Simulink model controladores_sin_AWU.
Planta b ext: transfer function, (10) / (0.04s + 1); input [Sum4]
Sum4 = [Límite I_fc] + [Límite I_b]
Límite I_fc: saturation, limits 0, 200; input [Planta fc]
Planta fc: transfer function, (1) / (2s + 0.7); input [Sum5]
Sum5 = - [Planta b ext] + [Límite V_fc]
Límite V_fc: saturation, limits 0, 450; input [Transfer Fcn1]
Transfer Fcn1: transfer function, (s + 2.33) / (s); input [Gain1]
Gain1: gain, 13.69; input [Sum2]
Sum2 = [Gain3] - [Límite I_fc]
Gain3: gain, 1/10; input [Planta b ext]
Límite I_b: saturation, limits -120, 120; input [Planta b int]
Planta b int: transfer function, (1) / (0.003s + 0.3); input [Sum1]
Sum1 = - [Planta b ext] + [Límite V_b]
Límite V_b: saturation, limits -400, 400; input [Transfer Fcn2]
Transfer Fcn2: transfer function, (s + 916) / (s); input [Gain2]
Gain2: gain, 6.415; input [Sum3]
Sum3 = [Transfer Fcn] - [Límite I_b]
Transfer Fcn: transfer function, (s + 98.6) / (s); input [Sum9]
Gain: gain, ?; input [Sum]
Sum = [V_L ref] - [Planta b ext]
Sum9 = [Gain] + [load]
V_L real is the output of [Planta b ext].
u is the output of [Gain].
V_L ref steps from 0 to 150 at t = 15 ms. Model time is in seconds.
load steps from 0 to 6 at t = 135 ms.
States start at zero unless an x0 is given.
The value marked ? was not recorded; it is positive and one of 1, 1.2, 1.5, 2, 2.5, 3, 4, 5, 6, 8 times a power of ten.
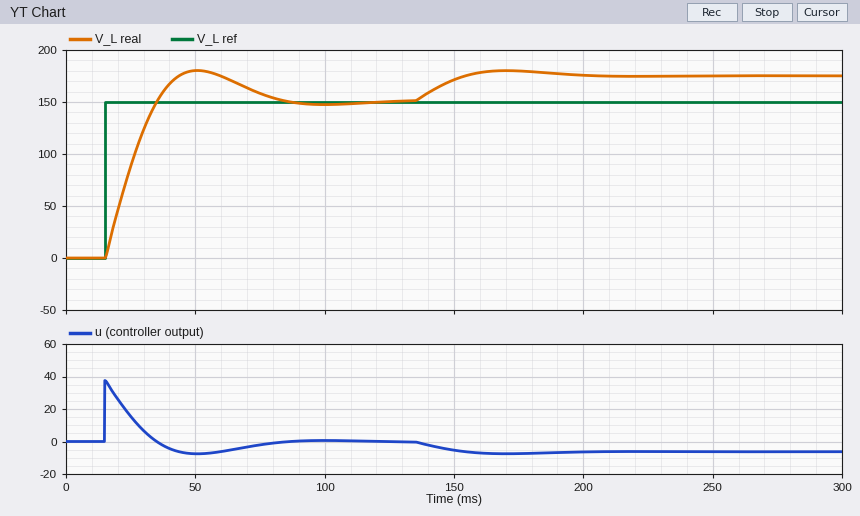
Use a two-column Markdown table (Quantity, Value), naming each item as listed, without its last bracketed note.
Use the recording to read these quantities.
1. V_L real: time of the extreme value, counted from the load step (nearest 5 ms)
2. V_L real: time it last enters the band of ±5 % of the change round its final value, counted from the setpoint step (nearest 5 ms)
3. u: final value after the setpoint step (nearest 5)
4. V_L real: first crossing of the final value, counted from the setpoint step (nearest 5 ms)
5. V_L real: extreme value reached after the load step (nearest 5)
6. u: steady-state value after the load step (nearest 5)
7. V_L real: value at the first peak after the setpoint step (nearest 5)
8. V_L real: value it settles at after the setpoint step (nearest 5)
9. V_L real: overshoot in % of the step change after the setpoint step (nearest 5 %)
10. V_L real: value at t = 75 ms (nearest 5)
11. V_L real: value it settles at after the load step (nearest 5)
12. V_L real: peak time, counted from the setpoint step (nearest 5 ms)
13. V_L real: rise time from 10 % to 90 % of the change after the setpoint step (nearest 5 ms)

| Quantity | Value |
|---|---|
| V_L real: time of the extreme value, counted from the load step | 35 ms |
| V_L real: time it last enters the band of ±5 % of the change round its final value, counted from the setpoint step | 60 ms |
| u: final value after the setpoint step | 0 |
| V_L real: first crossing of the final value, counted from the setpoint step | 20 ms |
| V_L real: extreme value reached after the load step | 180 |
| u: steady-state value after the load step | -5 |
| V_L real: value at the first peak after the setpoint step | 180 |
| V_L real: value it settles at after the setpoint step | 150 |
| V_L real: overshoot in % of the step change after the setpoint step | 20 % |
| V_L real: value at t = 75 ms | 160 |
| V_L real: value it settles at after the load step | 175 |
| V_L real: peak time, counted from the setpoint step | 35 ms |
| V_L real: rise time from 10 % to 90 % of the change after the setpoint step | 15 ms |
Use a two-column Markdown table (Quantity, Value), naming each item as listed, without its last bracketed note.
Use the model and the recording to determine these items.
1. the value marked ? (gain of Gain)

| Quantity | Value |
|---|---|
| the value marked ? | 0.25 |
